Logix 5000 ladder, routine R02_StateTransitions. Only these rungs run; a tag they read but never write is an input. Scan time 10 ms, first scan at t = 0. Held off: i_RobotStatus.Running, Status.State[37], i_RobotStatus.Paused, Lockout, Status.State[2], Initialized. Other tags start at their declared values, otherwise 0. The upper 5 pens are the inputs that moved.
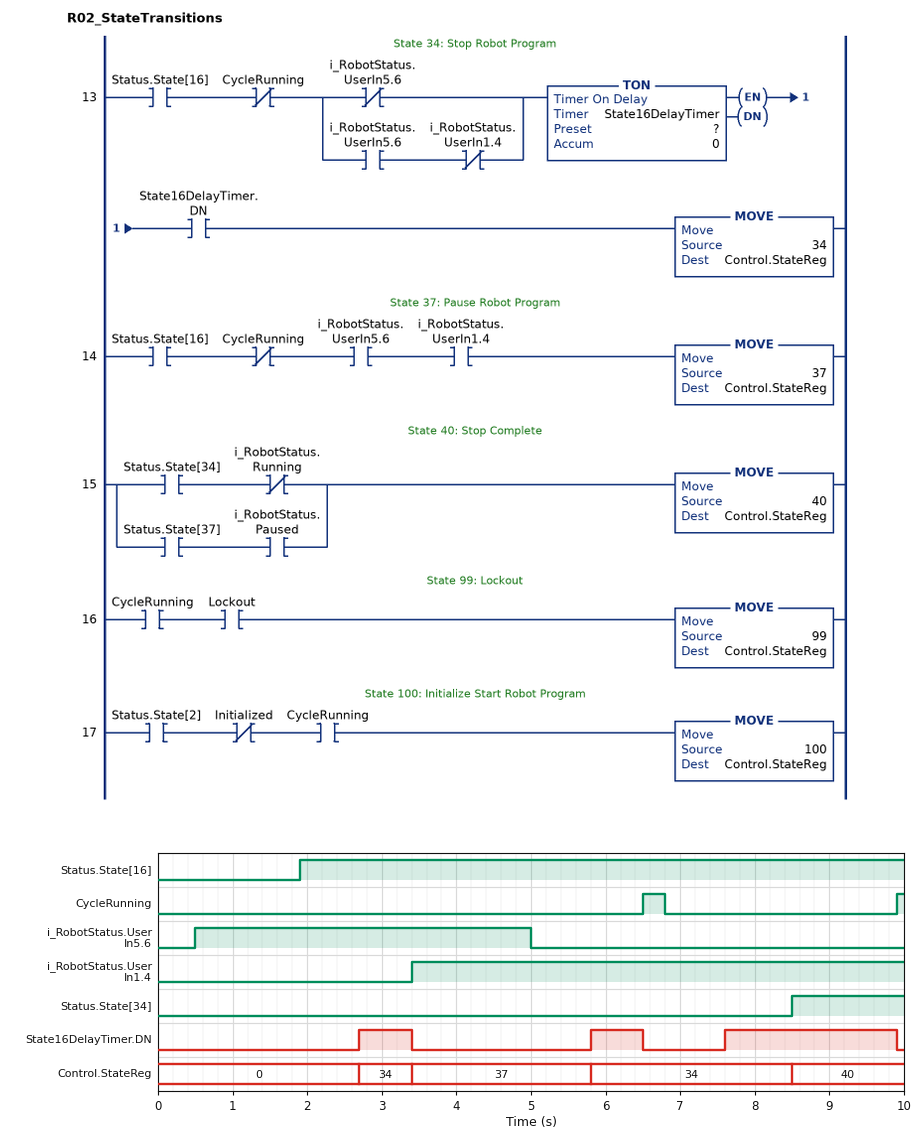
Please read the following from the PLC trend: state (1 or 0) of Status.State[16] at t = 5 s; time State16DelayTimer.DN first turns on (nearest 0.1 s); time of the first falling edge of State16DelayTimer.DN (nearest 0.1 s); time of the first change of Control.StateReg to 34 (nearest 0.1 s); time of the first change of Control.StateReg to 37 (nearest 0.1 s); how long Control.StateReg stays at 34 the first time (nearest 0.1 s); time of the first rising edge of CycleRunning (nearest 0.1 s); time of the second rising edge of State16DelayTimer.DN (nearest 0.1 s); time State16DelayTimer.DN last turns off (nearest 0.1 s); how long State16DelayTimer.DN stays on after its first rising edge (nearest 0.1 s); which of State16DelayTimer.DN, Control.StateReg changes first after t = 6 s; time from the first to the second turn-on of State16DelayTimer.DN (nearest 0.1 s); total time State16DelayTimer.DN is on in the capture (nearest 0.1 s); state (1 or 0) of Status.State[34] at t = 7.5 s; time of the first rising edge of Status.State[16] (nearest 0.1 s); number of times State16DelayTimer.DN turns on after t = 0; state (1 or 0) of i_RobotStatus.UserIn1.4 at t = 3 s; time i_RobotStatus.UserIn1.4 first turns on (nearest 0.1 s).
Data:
1
2.7 s
3.4 s
2.7 s
3.4 s
0.7 s
6.5 s
5.8 s
9.9 s
0.7 s
State16DelayTimer.DN
3.1 s
3.7 s
0
1.9 s
3
0
3.4 s
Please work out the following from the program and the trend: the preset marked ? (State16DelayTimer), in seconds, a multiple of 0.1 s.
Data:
0.8 s
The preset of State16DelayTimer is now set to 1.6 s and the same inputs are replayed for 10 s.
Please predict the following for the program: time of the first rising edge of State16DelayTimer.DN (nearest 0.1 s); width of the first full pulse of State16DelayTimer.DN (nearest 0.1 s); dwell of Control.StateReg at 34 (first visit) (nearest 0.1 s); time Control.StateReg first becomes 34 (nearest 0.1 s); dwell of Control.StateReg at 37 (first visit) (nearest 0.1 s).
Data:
8.4 s
1.5 s
0.1 s
8.4 s
5.0 s
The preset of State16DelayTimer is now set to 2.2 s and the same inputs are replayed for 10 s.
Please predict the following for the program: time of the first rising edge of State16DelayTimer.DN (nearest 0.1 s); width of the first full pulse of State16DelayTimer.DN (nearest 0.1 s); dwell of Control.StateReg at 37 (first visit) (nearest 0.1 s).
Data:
9.0 s
0.9 s
5.1 s
